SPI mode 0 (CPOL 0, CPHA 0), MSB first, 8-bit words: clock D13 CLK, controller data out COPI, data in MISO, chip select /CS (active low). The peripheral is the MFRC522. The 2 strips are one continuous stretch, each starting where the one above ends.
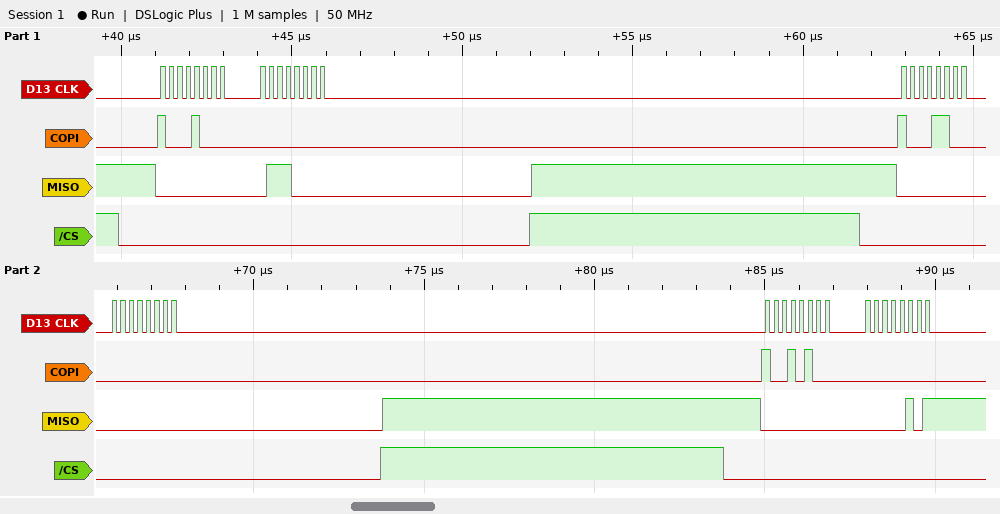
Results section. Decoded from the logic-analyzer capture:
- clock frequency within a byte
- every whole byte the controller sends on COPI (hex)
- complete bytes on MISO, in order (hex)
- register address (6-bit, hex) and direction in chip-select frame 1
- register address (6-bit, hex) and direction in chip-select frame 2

4 MHz
0x88 0x00 0x8C 0x00 0x94 0x00
0x00 0x70 0x00 0x00 0x00 0x05
0x04 read
0x06 read
